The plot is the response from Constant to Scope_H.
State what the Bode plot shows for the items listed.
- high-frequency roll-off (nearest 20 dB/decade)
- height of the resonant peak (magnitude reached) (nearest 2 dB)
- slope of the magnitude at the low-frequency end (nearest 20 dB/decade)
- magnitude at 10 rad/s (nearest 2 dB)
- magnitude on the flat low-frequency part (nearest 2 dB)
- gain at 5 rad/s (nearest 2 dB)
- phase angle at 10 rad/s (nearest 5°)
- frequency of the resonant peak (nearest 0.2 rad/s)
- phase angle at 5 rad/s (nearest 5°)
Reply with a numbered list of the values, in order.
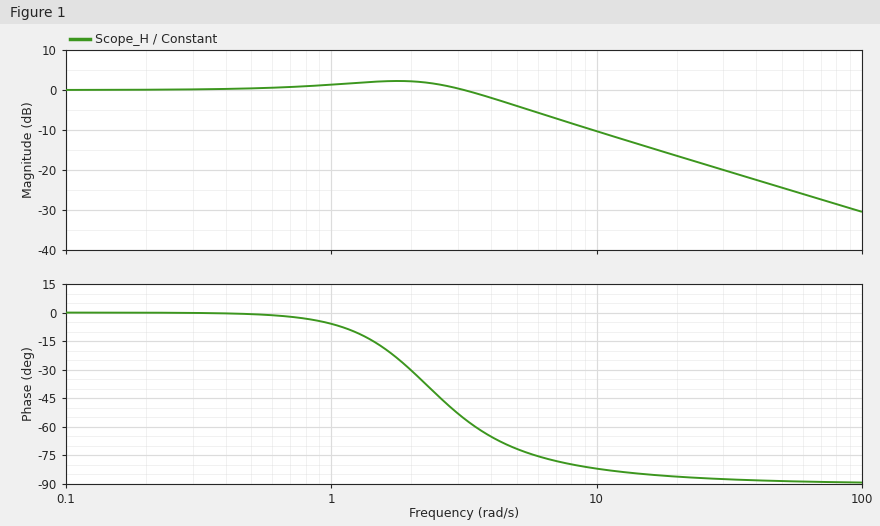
1. -20 dB/decade
2. 2 dB
3. 0 dB/decade
4. -10 dB
5. 0 dB
6. -4 dB
7. -80°
8. 1.8 rad/s
9. -70°
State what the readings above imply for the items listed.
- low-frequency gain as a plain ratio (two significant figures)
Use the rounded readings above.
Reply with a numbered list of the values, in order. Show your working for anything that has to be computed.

1. 10^(0 / 20) = 1.0
